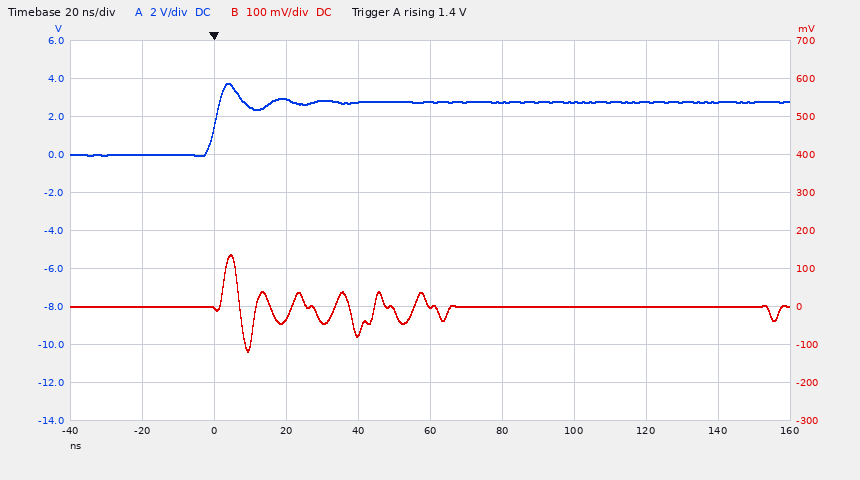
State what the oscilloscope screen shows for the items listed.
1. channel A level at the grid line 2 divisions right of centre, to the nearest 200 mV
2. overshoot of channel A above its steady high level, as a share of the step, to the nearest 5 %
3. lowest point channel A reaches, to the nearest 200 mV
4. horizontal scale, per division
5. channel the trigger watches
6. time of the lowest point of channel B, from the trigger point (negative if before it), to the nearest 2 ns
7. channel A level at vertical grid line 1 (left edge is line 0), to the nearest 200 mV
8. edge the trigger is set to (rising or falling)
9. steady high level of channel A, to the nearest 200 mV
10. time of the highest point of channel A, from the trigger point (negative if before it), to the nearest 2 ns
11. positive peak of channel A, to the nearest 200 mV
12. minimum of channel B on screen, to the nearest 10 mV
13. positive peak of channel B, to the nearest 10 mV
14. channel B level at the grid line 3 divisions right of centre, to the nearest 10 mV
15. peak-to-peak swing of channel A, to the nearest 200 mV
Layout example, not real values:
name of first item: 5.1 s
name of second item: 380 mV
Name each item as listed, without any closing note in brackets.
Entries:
channel A level at the grid line 2 divisions right of centre, to the nearest 200 mV: 2.8 V
overshoot of channel A above its steady high level, as a share of the step, to the nearest 5 %: 35 %
lowest point channel A reaches, to the nearest 200 mV: 0.0 V
horizontal scale, per division: 20 ns
channel the trigger watches: channel A
time of the lowest point of channel B, from the trigger point (negative if before it), to the nearest 2 ns: +10 ns
channel A level at vertical grid line 1 (left edge is line 0), to the nearest 200 mV: 0.0 V
edge the trigger is set to: rising
steady high level of channel A, to the nearest 200 mV: 2.8 V
time of the highest point of channel A, from the trigger point (negative if before it), to the nearest 2 ns: +4 ns
positive peak of channel A, to the nearest 200 mV: 3.8 V
minimum of channel B on screen, to the nearest 10 mV: -120 mV
positive peak of channel B, to the nearest 10 mV: 140 mV
channel B level at the grid line 3 divisions right of centre, to the nearest 10 mV: 0 mV
peak-to-peak swing of channel A, to the nearest 200 mV: 3.8 V
